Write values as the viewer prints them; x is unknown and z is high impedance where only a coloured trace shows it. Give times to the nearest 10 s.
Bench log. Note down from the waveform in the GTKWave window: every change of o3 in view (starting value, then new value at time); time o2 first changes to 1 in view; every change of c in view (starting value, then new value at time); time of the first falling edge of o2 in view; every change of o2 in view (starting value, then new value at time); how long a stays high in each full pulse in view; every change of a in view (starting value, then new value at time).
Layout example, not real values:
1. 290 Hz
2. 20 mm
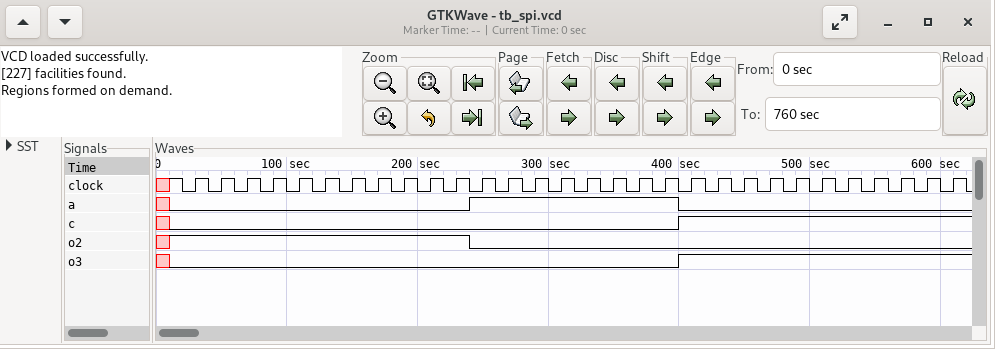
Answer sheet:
1. x, 0 at 10 s, 1 at 400 s
2. 10 s
3. x, 0 at 10 s, 1 at 400 s
4. 240 s
5. x, 1 at 10 s, 0 at 240 s
6. 160 s
7. x, 0 at 10 s, 1 at 240 s, 0 at 400 s
